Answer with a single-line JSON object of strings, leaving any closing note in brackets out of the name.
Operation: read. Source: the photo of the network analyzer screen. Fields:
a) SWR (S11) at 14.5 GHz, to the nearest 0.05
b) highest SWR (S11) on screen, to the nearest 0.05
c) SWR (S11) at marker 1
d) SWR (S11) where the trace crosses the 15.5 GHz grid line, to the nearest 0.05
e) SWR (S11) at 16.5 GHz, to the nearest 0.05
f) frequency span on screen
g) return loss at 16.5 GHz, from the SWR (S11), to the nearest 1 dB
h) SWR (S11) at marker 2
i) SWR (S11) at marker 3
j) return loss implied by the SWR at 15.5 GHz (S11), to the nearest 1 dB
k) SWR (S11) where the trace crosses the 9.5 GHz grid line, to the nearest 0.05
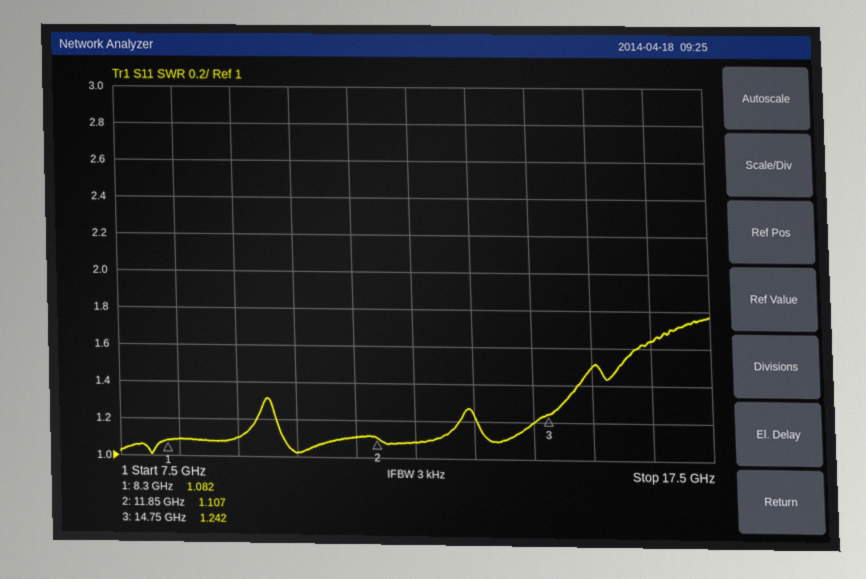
{"SWR (S11) at 14.5 GHz, to the nearest 0.05": "1.20", "highest SWR (S11) on screen, to the nearest 0.05": "1.75", "SWR (S11) at marker 1": "1.082", "SWR (S11) where the trace crosses the 15.5 GHz grid line, to the nearest 0.05": "1.50", "SWR (S11) at 16.5 GHz, to the nearest 0.05": "1.65", "frequency span on screen": "10 GHz", "return loss at 16.5 GHz, from the SWR (S11), to the nearest 1 dB": "12 dB", "SWR (S11) at marker 2": "1.107", "SWR (S11) at marker 3": "1.242", "return loss implied by the SWR at 15.5 GHz (S11), to the nearest 1 dB": "14 dB", "SWR (S11) where the trace crosses the 9.5 GHz grid line, to the nearest 0.05": "1.10"}
